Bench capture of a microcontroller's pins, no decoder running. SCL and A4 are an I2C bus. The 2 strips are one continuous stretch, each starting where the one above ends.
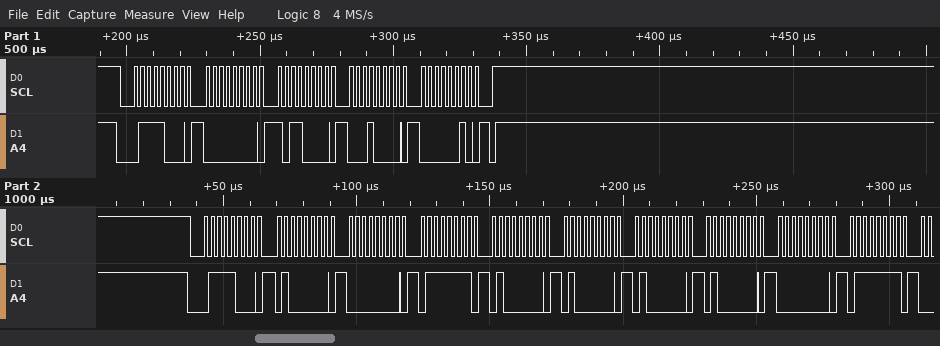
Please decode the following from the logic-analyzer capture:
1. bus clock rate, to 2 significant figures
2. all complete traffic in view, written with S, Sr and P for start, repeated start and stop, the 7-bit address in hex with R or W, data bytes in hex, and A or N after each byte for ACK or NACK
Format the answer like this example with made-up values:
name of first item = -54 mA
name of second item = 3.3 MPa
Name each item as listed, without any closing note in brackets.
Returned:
bus clock rate, to 2 significant figures = 400 kHz
all complete traffic in view, written with S, Sr and P for start, repeated start and stop, the 7-bit address in hex with R or W, data bytes in hex, and A or N after each byte for ACK or NACK = S 3CW A 00 A B0 A 10 A 02 A P S 3CW A 40 A 00 A 7F A 40 A 40 A 40 A 40 A 00 A 7F A
